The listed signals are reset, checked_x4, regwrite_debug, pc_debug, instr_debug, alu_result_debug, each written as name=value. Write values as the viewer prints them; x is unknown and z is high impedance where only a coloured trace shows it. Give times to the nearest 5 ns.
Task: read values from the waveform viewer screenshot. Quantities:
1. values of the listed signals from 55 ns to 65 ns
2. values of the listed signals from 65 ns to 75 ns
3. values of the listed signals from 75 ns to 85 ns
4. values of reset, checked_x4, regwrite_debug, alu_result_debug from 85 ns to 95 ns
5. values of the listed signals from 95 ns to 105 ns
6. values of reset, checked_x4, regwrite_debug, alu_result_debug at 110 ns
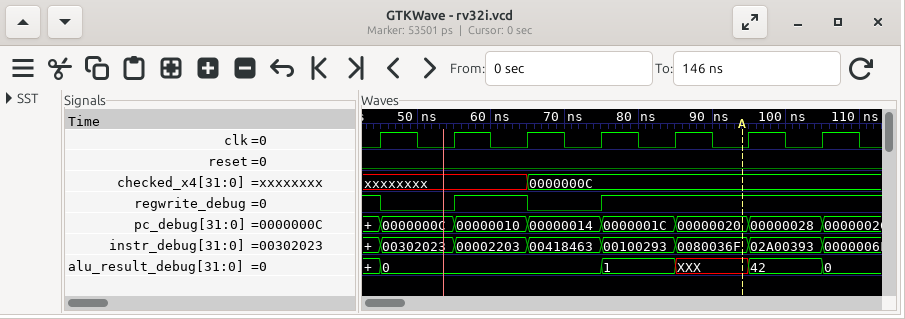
reset=0, checked_x4=xxxxxxxx, regwrite_debug=1, pc_debug=00000010, instr_debug=00002203, alu_result_debug=0
reset=0, checked_x4=0000000C, regwrite_debug=0, pc_debug=00000014, instr_debug=00418463, alu_result_debug=0
reset=0, checked_x4=0000000C, regwrite_debug=1, pc_debug=0000001C, instr_debug=00100293, alu_result_debug=1
reset=0, checked_x4=0000000C, regwrite_debug=1, alu_result_debug=XXX
reset=0, checked_x4=0000000C, regwrite_debug=1, pc_debug=00000028, instr_debug=02A00393, alu_result_debug=42
reset=0, checked_x4=0000000C, regwrite_debug=1, alu_result_debug=0
